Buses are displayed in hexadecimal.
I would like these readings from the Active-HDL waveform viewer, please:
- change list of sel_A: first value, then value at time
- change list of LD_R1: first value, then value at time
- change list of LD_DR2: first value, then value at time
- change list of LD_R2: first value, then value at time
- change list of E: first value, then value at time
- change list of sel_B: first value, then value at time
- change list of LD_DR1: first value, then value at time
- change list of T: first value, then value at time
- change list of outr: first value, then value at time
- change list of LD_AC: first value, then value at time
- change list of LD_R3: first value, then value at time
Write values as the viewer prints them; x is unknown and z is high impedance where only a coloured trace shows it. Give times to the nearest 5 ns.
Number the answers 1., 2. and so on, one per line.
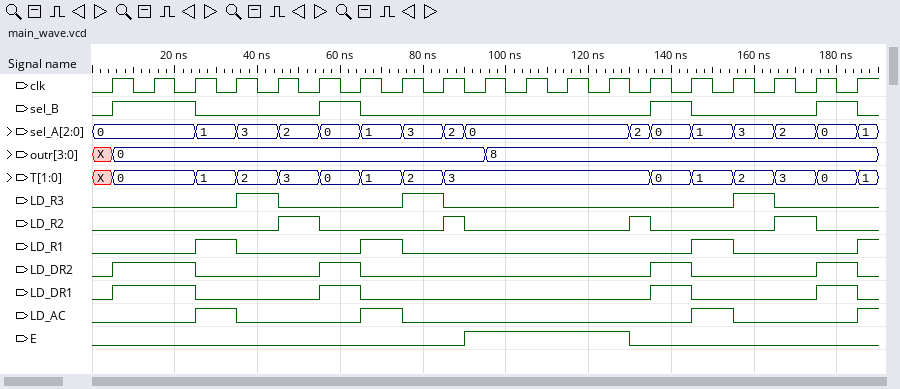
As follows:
1. 0, 1 at 25 ns, 3 at 35 ns, 2 at 45 ns, 0 at 55 ns, 1 at 65 ns, 3 at 75 ns, 2 at 85 ns, 0 at 90 ns, 2 at 130 ns, 0 at 135 ns, 1 at 145 ns, 3 at 155 ns, 2 at 165 ns, 0 at 175 ns, 1 at 185 ns
2. 0, 1 at 25 ns, 0 at 35 ns, 1 at 65 ns, 0 at 75 ns, 1 at 145 ns, 0 at 155 ns, 1 at 185 ns
3. 0, 1 at 5 ns, 0 at 25 ns, 1 at 55 ns, 0 at 65 ns, 1 at 135 ns, 0 at 145 ns, 1 at 175 ns, 0 at 185 ns
4. 0, 1 at 45 ns, 0 at 55 ns, 1 at 85 ns, 0 at 90 ns, 1 at 130 ns, 0 at 135 ns, 1 at 165 ns, 0 at 175 ns
5. 0, 1 at 90 ns, 0 at 130 ns
6. 0, 1 at 5 ns, 0 at 25 ns, 1 at 55 ns, 0 at 65 ns, 1 at 135 ns, 0 at 145 ns, 1 at 175 ns, 0 at 185 ns
7. 0, 1 at 5 ns, 0 at 25 ns, 1 at 55 ns, 0 at 65 ns, 1 at 135 ns, 0 at 145 ns, 1 at 175 ns, 0 at 185 ns
8. X, 0 at 5 ns, 1 at 25 ns, 2 at 35 ns, 3 at 45 ns, 0 at 55 ns, 1 at 65 ns, 2 at 75 ns, 3 at 85 ns, 0 at 135 ns, 1 at 145 ns, 2 at 155 ns, 3 at 165 ns, 0 at 175 ns, 1 at 185 ns
9. X, 0 at 5 ns, 8 at 95 ns
10. 0, 1 at 25 ns, 0 at 35 ns, 1 at 65 ns, 0 at 75 ns, 1 at 145 ns, 0 at 155 ns, 1 at 185 ns
11. 0, 1 at 35 ns, 0 at 45 ns, 1 at 75 ns, 0 at 85 ns, 1 at 155 ns, 0 at 165 ns
